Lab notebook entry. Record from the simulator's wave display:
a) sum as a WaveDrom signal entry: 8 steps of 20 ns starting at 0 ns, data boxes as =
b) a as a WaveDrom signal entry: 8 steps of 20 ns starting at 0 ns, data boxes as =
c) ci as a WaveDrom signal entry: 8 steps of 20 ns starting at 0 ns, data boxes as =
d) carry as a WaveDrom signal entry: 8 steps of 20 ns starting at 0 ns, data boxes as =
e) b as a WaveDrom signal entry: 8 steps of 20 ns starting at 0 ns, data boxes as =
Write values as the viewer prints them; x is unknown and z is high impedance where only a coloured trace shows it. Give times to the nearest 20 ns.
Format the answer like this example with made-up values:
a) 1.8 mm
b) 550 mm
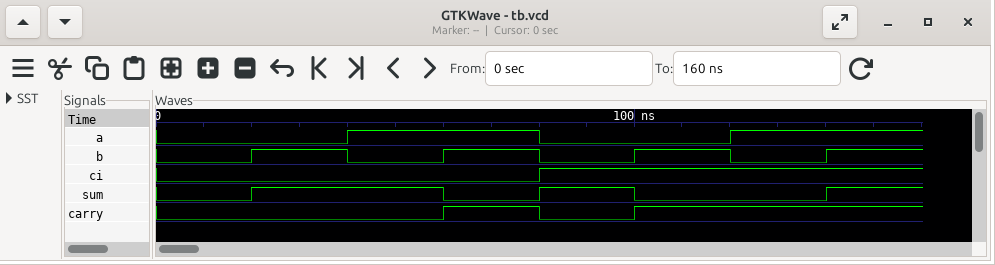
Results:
a) {name: 'sum', wave: '01.010.1'}
b) {name: 'a', wave: '0.1.0.1.'}
c) {name: 'ci', wave: '0...1...'}
d) {name: 'carry', wave: '0..101..'}
e) {name: 'b', wave: '01010101'}
